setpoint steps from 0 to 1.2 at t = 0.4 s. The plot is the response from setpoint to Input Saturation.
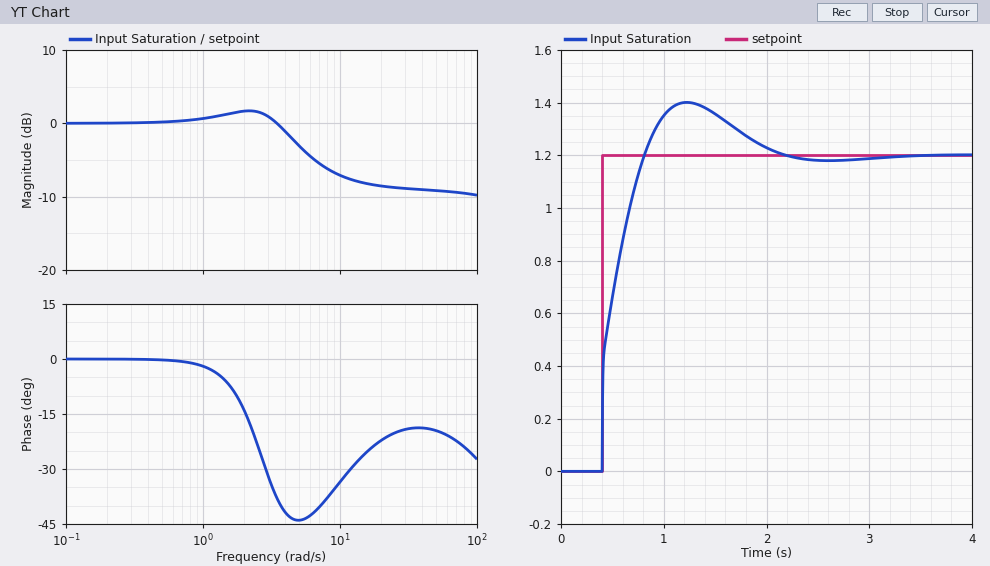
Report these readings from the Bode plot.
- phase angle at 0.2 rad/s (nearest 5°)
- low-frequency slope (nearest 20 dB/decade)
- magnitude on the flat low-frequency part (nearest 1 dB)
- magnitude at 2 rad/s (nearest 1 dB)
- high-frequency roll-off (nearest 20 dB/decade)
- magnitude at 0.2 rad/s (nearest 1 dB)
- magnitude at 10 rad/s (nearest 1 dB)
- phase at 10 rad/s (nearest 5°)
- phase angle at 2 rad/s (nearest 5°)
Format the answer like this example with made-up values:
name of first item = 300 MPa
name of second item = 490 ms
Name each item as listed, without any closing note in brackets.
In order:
phase angle at 0.2 rad/s = 0°
low-frequency slope = 0 dB/decade
magnitude on the flat low-frequency part = 0 dB
magnitude at 2 rad/s = 2 dB
high-frequency roll-off = 0 dB/decade
magnitude at 0.2 rad/s = 0 dB
magnitude at 10 rad/s = -7 dB
phase at 10 rad/s = -35°
phase angle at 2 rad/s = -15°
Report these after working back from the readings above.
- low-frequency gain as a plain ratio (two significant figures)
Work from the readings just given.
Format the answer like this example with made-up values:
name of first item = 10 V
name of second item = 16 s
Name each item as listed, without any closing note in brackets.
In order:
low-frequency gain as a plain ratio = 1.0
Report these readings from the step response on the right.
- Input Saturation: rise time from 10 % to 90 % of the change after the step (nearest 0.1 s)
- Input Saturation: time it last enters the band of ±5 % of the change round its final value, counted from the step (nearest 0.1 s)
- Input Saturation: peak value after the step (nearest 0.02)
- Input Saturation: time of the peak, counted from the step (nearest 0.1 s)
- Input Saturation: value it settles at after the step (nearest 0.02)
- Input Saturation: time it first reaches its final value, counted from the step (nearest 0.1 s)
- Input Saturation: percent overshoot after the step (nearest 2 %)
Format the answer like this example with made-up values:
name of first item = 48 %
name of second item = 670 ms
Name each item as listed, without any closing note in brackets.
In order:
Input Saturation: rise time from 10 % to 90 % of the change after the step = 0.3 s
Input Saturation: time it last enters the band of ±5 % of the change round its final value, counted from the step = 1.5 s
Input Saturation: peak value after the step = 1.40
Input Saturation: time of the peak, counted from the step = 0.8 s
Input Saturation: value it settles at after the step = 1.20
Input Saturation: time it first reaches its final value, counted from the step = 0.4 s
Input Saturation: percent overshoot after the step = 16 %
